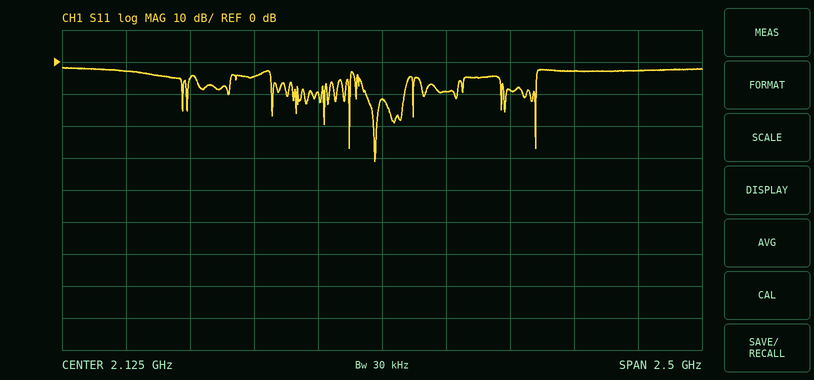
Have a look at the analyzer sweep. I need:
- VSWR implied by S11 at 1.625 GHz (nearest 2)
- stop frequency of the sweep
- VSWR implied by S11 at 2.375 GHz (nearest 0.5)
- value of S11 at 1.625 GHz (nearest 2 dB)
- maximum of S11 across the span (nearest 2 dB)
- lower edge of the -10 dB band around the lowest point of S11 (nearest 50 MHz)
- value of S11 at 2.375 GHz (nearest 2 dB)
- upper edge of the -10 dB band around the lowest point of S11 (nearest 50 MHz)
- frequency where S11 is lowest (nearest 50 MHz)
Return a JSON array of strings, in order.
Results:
["4", "3.375 GHz", "2.0", "-4 dB", "-2 dB", "2.05 GHz", "-10 dB", "2.20 GHz", "2.10 GHz"]
